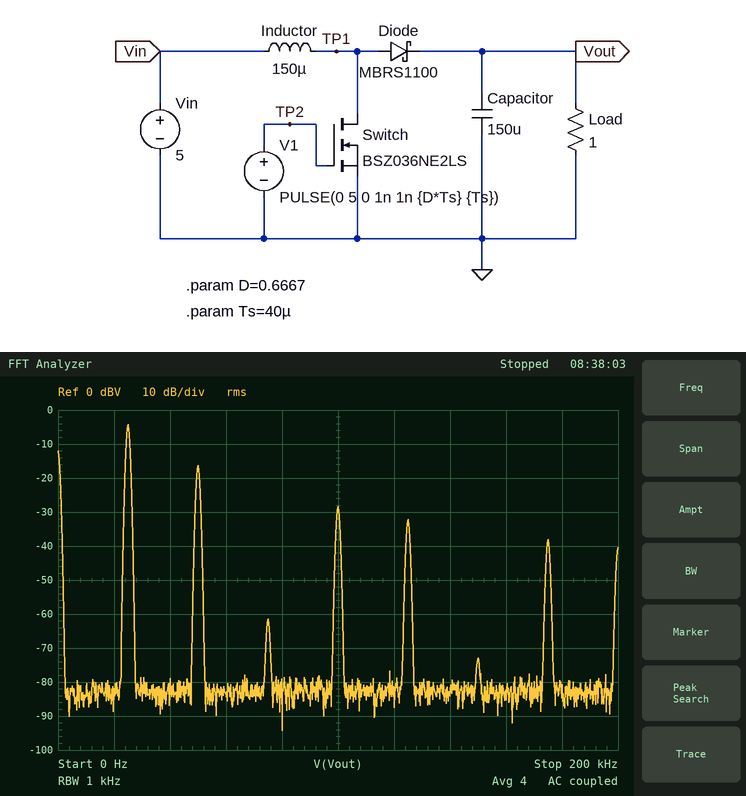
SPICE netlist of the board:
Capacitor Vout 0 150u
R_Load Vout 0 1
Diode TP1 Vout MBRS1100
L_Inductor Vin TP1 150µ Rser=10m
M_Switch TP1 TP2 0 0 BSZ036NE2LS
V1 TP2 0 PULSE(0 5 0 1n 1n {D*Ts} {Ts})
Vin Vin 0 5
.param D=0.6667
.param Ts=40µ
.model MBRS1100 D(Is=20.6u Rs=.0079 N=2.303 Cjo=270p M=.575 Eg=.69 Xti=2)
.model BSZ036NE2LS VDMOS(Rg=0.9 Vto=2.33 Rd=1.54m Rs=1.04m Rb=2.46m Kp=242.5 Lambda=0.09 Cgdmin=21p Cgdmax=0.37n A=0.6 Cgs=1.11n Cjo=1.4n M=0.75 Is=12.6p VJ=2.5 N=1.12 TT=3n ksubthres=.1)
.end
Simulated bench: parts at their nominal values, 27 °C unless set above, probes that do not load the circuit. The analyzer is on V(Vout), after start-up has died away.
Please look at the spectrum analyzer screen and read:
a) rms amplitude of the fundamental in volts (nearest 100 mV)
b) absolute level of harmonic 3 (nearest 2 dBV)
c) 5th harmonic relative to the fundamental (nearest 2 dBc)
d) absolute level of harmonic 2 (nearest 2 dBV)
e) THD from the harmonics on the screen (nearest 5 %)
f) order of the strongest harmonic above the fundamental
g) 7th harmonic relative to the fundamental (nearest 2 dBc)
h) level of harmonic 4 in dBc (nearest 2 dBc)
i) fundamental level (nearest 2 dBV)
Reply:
600 mV
-62 dBV
-28 dBc
-16 dBV
25 %
2
-34 dBc
-24 dBc
-4 dBV
